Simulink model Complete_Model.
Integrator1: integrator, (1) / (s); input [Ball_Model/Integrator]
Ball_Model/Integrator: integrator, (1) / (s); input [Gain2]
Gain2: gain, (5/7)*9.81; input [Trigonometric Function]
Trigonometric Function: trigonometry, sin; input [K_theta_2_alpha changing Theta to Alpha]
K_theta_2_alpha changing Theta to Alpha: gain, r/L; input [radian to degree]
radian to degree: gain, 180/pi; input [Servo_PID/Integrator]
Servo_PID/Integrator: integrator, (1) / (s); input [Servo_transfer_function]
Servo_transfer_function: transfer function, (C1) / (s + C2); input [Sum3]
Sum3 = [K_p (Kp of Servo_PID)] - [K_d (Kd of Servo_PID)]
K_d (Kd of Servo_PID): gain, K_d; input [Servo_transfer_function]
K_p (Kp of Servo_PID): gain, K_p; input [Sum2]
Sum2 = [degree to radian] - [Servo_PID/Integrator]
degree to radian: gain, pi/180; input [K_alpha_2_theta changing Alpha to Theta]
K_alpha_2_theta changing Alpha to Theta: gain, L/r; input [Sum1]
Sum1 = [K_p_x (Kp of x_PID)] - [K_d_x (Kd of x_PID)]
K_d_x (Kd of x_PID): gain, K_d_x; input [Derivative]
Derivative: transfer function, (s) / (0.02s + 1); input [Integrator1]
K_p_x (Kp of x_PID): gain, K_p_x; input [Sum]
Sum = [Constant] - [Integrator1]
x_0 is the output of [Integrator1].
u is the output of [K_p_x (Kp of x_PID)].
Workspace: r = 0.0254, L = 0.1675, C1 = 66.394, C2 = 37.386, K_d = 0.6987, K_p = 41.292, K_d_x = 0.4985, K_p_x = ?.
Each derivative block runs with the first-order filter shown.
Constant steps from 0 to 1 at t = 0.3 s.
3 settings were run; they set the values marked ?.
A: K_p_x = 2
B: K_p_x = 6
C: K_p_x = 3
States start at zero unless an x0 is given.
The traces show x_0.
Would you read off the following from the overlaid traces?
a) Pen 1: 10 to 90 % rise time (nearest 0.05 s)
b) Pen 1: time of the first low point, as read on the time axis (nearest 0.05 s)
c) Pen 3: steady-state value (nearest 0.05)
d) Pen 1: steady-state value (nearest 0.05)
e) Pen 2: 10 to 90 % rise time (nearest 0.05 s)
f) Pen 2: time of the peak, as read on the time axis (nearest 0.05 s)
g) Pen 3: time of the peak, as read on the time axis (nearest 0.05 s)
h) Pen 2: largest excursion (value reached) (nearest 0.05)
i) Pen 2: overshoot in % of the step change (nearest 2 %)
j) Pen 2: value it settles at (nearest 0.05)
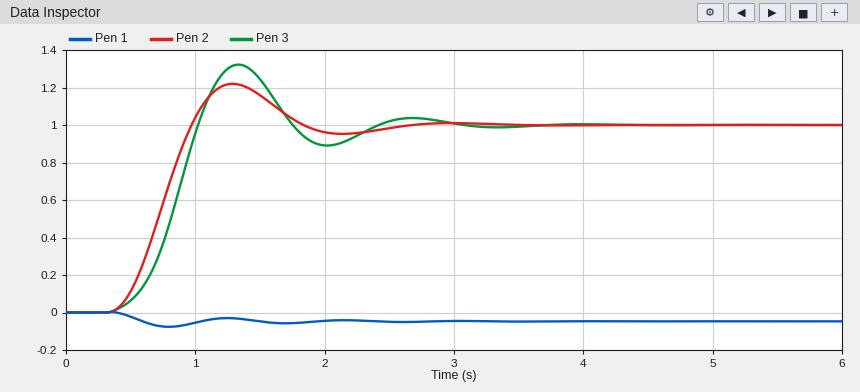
0.15 s
0.80 s
1.00
-0.05
0.40 s
1.30 s
1.35 s
1.20
22 %
1.00
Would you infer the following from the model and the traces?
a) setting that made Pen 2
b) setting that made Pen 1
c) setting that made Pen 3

A
B
C
